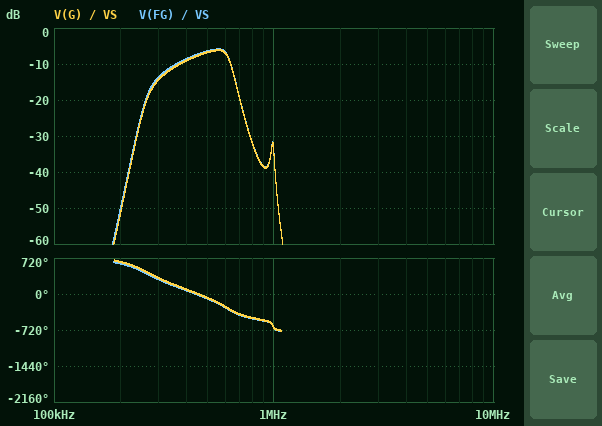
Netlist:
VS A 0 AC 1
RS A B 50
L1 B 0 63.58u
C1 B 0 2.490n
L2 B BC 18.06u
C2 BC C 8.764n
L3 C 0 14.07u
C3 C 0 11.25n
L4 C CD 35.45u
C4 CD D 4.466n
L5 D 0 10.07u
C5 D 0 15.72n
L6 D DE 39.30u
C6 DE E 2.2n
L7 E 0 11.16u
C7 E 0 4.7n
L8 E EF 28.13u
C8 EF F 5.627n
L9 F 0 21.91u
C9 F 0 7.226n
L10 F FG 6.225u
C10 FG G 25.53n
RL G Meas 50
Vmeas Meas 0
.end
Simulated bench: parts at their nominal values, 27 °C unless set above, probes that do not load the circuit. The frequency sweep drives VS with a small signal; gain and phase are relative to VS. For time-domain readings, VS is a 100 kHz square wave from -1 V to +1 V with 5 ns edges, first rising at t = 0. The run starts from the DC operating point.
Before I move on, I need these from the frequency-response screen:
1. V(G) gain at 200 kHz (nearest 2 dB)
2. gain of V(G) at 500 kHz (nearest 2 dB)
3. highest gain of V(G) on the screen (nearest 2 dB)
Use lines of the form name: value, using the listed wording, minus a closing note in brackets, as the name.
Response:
V(G) gain at 200 kHz: -52 dB
gain of V(G) at 500 kHz: -6 dB
highest gain of V(G) on the screen: -6 dB
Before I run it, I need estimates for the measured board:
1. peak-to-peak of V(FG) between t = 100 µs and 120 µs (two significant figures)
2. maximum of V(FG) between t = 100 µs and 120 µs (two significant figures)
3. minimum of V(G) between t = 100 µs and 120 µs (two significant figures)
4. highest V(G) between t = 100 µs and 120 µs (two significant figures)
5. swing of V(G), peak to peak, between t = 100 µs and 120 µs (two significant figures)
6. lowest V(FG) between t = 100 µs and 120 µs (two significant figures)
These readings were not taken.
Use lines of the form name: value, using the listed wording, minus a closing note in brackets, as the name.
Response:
peak-to-peak of V(FG) between t = 100 µs and 120 µs: 440 mV
maximum of V(FG) between t = 100 µs and 120 µs: 220 mV
minimum of V(G) between t = 100 µs and 120 µs: -200 mV
highest V(G) between t = 100 µs and 120 µs: 200 mV
swing of V(G), peak to peak, between t = 100 µs and 120 µs: 410 mV
lowest V(FG) between t = 100 µs and 120 µs: -220 mV
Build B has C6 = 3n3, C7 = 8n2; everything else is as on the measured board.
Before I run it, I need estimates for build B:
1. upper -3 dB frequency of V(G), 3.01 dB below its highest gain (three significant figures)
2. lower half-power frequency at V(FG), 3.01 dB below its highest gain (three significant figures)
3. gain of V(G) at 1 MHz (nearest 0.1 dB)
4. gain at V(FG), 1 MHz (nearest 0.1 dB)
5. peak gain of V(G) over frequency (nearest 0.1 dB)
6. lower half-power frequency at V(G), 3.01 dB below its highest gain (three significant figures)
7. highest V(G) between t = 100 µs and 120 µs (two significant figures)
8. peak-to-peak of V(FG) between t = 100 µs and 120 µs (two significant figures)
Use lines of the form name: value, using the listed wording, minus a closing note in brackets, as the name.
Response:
upper -3 dB frequency of V(G), 3.01 dB below its highest gain: 615 kHz
lower half-power frequency at V(FG), 3.01 dB below its highest gain: 270 kHz
gain of V(G) at 1 MHz: -61.8 dB
gain at V(FG), 1 MHz: -61.7 dB
peak gain of V(G) over frequency: -6.2 dB
lower half-power frequency at V(G), 3.01 dB below its highest gain: 273 kHz
highest V(G) between t = 100 µs and 120 µs: 310 mV
peak-to-peak of V(FG) between t = 100 µs and 120 µs: 660 mV
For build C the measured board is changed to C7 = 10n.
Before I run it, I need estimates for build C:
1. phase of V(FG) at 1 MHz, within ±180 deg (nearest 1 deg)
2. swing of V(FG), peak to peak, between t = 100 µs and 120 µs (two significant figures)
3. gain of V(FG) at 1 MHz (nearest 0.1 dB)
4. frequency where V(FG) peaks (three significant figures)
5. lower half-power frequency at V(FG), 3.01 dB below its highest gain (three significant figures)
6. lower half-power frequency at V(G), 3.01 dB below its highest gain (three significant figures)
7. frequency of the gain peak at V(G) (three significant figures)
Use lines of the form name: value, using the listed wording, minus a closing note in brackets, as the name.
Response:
phase of V(FG) at 1 MHz, within ±180 deg: -7 deg
swing of V(FG), peak to peak, between t = 100 µs and 120 µs: 530 mV
gain of V(FG) at 1 MHz: -63.7 dB
frequency where V(FG) peaks: 518 kHz
lower half-power frequency at V(FG), 3.01 dB below its highest gain: 336 kHz
lower half-power frequency at V(G), 3.01 dB below its highest gain: 344 kHz
frequency of the gain peak at V(G): 522 kHz
